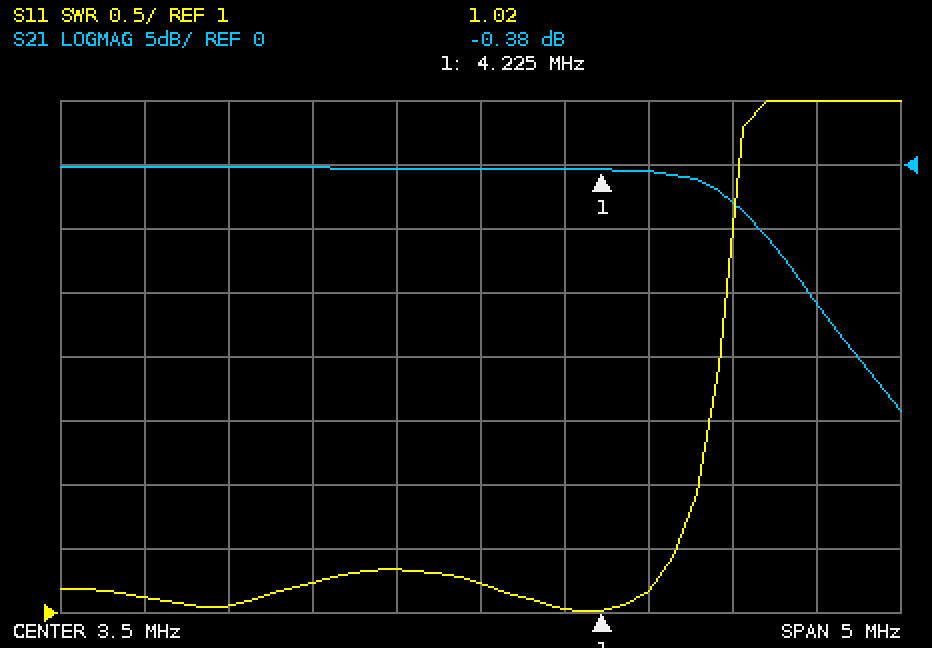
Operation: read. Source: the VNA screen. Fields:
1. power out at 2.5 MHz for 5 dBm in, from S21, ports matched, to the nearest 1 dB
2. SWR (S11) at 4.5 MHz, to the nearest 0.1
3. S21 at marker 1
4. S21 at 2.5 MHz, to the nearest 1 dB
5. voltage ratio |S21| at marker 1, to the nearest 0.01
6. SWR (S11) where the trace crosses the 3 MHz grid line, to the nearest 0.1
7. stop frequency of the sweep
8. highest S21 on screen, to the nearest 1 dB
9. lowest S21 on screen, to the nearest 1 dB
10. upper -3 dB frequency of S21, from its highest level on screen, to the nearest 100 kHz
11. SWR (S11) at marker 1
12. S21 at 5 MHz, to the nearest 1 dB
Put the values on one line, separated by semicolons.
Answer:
5 dBm; 1.2; -0.38 dB; 0 dB; 0.96; 1.3; 6 MHz; 0 dB; -19 dB; 5.0 MHz; 1.02; -3 dB
